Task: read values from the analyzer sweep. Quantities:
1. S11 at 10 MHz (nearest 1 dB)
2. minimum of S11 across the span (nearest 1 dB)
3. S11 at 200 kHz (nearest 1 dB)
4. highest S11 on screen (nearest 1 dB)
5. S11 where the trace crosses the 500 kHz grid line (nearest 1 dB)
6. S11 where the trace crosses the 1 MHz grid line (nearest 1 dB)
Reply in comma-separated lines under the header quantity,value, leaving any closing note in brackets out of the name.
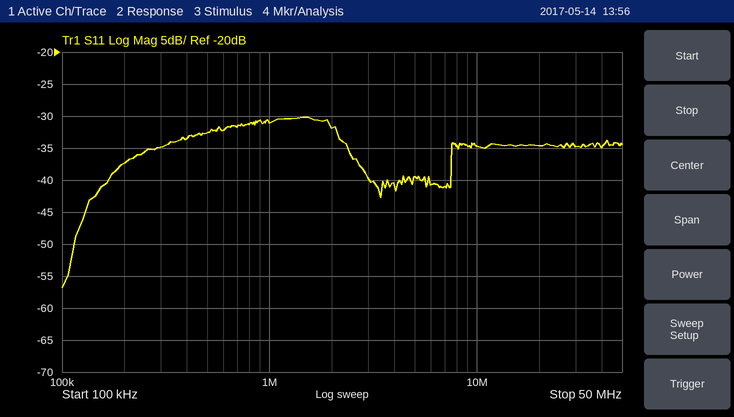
quantity,value
S11 at 10 MHz,-35 dB
minimum of S11 across the span,-57 dB
S11 at 200 kHz,-37 dB
highest S11 on screen,-30 dB
S11 where the trace crosses the 500 kHz grid line,-33 dB
S11 where the trace crosses the 1 MHz grid line,-31 dB
